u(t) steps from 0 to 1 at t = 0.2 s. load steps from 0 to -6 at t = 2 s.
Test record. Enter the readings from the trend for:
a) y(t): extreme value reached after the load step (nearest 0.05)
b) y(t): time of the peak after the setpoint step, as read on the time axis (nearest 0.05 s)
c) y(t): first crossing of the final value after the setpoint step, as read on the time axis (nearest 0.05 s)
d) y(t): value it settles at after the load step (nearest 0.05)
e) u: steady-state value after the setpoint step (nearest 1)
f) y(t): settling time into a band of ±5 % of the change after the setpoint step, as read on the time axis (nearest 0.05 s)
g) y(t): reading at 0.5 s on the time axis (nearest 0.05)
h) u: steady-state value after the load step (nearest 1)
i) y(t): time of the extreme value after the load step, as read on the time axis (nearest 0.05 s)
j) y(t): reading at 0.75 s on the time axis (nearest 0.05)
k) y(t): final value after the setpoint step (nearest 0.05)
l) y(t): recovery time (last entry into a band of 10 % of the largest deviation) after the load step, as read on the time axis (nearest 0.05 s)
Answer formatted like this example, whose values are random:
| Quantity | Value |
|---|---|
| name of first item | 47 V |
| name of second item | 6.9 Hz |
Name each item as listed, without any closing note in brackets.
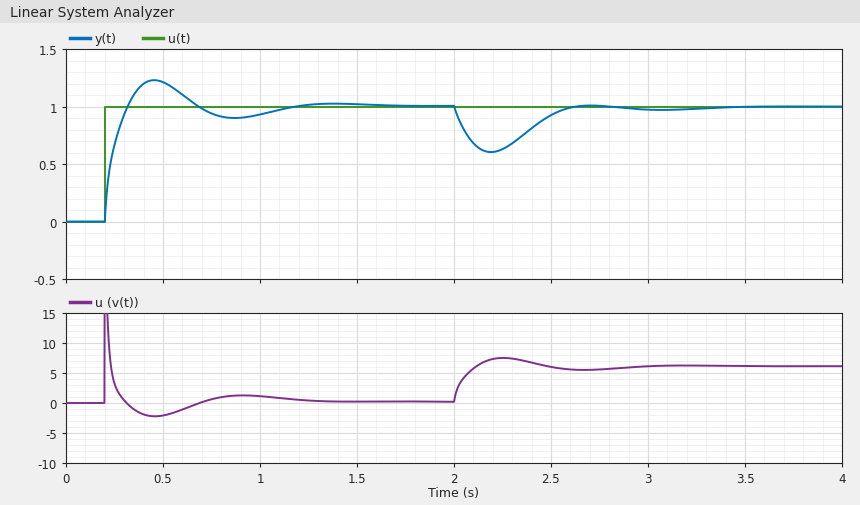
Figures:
| Quantity | Value |
|---|---|
| y(t): extreme value reached after the load step | 0.60 |
| y(t): time of the peak after the setpoint step, as read on the time axis | 0.45 s |
| y(t): first crossing of the final value after the setpoint step, as read on the time axis | 0.30 s |
| y(t): value it settles at after the load step | 1.00 |
| u: steady-state value after the setpoint step | 0 |
| y(t): settling time into a band of ±5 % of the change after the setpoint step, as read on the time axis | 1.05 s |
| y(t): reading at 0.5 s on the time axis | 1.20 |
| u: steady-state value after the load step | 6 |
| y(t): time of the extreme value after the load step, as read on the time axis | 2.20 s |
| y(t): reading at 0.75 s on the time axis | 0.95 |
| y(t): final value after the setpoint step | 1.00 |
| y(t): recovery time (last entry into a band of 10 % of the largest deviation) after the load step, as read on the time axis | 2.55 s |
